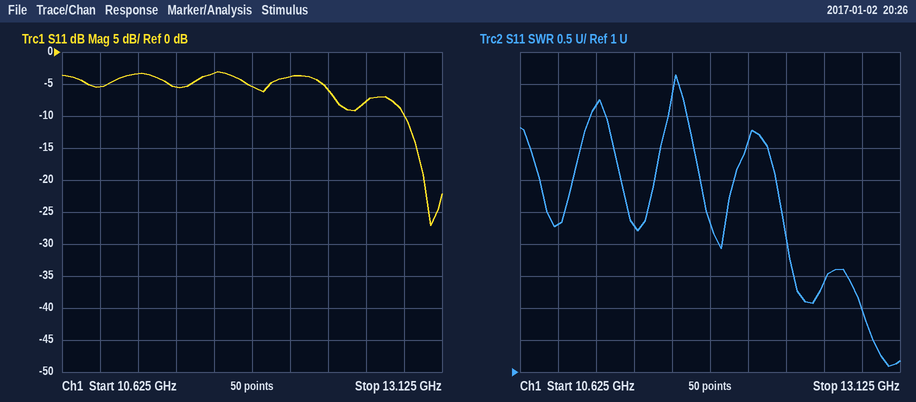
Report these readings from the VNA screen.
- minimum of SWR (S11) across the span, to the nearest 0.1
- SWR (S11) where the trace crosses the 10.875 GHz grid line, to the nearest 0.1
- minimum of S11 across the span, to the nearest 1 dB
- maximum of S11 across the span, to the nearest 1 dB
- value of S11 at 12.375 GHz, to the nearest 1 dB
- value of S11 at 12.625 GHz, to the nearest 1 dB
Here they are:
1.1
3.3
-27 dB
-3 dB
-6 dB
-8 dB
